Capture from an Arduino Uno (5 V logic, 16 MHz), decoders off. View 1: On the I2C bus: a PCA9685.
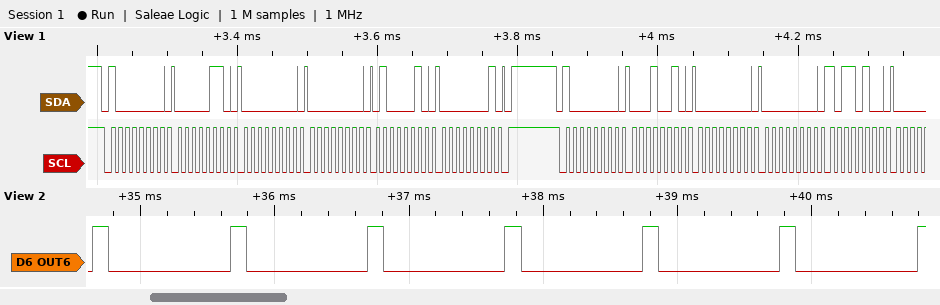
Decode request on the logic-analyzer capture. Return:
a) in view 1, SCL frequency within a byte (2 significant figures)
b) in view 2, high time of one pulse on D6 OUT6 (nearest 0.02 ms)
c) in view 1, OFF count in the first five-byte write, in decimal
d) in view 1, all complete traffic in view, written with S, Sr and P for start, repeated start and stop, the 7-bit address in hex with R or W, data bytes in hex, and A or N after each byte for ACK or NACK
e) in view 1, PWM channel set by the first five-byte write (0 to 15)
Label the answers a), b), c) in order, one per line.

a) 100 kHz
b) 0.12 ms
c) 322
d) S 40W A 06 A 00 A 00 A 42 A 01 A P S 40W A 12 A 00 A 00 A B4 A
e) 0
